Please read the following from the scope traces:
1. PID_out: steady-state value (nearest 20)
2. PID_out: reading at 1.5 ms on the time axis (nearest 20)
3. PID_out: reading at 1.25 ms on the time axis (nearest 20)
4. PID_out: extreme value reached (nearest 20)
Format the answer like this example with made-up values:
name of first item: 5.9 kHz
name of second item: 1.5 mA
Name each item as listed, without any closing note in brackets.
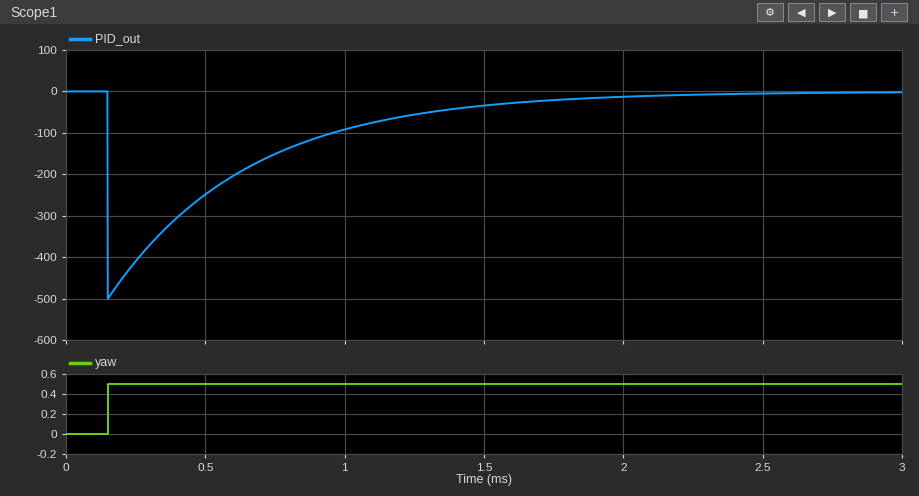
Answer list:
PID_out: steady-state value: 0
PID_out: reading at 1.5 ms on the time axis: -40
PID_out: reading at 1.25 ms on the time axis: -60
PID_out: extreme value reached: -500
